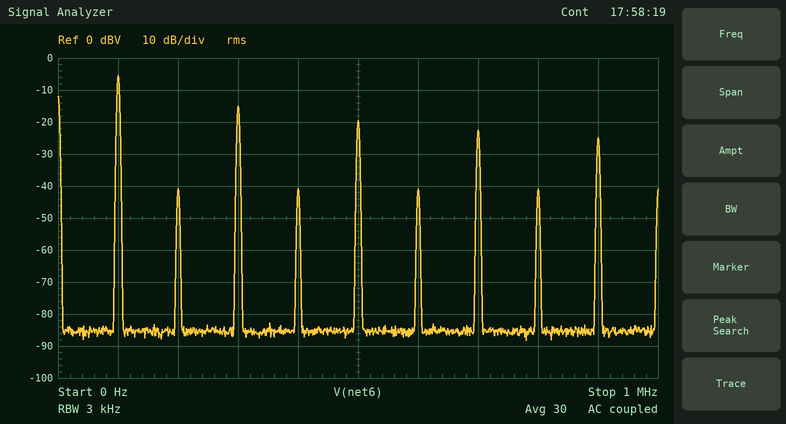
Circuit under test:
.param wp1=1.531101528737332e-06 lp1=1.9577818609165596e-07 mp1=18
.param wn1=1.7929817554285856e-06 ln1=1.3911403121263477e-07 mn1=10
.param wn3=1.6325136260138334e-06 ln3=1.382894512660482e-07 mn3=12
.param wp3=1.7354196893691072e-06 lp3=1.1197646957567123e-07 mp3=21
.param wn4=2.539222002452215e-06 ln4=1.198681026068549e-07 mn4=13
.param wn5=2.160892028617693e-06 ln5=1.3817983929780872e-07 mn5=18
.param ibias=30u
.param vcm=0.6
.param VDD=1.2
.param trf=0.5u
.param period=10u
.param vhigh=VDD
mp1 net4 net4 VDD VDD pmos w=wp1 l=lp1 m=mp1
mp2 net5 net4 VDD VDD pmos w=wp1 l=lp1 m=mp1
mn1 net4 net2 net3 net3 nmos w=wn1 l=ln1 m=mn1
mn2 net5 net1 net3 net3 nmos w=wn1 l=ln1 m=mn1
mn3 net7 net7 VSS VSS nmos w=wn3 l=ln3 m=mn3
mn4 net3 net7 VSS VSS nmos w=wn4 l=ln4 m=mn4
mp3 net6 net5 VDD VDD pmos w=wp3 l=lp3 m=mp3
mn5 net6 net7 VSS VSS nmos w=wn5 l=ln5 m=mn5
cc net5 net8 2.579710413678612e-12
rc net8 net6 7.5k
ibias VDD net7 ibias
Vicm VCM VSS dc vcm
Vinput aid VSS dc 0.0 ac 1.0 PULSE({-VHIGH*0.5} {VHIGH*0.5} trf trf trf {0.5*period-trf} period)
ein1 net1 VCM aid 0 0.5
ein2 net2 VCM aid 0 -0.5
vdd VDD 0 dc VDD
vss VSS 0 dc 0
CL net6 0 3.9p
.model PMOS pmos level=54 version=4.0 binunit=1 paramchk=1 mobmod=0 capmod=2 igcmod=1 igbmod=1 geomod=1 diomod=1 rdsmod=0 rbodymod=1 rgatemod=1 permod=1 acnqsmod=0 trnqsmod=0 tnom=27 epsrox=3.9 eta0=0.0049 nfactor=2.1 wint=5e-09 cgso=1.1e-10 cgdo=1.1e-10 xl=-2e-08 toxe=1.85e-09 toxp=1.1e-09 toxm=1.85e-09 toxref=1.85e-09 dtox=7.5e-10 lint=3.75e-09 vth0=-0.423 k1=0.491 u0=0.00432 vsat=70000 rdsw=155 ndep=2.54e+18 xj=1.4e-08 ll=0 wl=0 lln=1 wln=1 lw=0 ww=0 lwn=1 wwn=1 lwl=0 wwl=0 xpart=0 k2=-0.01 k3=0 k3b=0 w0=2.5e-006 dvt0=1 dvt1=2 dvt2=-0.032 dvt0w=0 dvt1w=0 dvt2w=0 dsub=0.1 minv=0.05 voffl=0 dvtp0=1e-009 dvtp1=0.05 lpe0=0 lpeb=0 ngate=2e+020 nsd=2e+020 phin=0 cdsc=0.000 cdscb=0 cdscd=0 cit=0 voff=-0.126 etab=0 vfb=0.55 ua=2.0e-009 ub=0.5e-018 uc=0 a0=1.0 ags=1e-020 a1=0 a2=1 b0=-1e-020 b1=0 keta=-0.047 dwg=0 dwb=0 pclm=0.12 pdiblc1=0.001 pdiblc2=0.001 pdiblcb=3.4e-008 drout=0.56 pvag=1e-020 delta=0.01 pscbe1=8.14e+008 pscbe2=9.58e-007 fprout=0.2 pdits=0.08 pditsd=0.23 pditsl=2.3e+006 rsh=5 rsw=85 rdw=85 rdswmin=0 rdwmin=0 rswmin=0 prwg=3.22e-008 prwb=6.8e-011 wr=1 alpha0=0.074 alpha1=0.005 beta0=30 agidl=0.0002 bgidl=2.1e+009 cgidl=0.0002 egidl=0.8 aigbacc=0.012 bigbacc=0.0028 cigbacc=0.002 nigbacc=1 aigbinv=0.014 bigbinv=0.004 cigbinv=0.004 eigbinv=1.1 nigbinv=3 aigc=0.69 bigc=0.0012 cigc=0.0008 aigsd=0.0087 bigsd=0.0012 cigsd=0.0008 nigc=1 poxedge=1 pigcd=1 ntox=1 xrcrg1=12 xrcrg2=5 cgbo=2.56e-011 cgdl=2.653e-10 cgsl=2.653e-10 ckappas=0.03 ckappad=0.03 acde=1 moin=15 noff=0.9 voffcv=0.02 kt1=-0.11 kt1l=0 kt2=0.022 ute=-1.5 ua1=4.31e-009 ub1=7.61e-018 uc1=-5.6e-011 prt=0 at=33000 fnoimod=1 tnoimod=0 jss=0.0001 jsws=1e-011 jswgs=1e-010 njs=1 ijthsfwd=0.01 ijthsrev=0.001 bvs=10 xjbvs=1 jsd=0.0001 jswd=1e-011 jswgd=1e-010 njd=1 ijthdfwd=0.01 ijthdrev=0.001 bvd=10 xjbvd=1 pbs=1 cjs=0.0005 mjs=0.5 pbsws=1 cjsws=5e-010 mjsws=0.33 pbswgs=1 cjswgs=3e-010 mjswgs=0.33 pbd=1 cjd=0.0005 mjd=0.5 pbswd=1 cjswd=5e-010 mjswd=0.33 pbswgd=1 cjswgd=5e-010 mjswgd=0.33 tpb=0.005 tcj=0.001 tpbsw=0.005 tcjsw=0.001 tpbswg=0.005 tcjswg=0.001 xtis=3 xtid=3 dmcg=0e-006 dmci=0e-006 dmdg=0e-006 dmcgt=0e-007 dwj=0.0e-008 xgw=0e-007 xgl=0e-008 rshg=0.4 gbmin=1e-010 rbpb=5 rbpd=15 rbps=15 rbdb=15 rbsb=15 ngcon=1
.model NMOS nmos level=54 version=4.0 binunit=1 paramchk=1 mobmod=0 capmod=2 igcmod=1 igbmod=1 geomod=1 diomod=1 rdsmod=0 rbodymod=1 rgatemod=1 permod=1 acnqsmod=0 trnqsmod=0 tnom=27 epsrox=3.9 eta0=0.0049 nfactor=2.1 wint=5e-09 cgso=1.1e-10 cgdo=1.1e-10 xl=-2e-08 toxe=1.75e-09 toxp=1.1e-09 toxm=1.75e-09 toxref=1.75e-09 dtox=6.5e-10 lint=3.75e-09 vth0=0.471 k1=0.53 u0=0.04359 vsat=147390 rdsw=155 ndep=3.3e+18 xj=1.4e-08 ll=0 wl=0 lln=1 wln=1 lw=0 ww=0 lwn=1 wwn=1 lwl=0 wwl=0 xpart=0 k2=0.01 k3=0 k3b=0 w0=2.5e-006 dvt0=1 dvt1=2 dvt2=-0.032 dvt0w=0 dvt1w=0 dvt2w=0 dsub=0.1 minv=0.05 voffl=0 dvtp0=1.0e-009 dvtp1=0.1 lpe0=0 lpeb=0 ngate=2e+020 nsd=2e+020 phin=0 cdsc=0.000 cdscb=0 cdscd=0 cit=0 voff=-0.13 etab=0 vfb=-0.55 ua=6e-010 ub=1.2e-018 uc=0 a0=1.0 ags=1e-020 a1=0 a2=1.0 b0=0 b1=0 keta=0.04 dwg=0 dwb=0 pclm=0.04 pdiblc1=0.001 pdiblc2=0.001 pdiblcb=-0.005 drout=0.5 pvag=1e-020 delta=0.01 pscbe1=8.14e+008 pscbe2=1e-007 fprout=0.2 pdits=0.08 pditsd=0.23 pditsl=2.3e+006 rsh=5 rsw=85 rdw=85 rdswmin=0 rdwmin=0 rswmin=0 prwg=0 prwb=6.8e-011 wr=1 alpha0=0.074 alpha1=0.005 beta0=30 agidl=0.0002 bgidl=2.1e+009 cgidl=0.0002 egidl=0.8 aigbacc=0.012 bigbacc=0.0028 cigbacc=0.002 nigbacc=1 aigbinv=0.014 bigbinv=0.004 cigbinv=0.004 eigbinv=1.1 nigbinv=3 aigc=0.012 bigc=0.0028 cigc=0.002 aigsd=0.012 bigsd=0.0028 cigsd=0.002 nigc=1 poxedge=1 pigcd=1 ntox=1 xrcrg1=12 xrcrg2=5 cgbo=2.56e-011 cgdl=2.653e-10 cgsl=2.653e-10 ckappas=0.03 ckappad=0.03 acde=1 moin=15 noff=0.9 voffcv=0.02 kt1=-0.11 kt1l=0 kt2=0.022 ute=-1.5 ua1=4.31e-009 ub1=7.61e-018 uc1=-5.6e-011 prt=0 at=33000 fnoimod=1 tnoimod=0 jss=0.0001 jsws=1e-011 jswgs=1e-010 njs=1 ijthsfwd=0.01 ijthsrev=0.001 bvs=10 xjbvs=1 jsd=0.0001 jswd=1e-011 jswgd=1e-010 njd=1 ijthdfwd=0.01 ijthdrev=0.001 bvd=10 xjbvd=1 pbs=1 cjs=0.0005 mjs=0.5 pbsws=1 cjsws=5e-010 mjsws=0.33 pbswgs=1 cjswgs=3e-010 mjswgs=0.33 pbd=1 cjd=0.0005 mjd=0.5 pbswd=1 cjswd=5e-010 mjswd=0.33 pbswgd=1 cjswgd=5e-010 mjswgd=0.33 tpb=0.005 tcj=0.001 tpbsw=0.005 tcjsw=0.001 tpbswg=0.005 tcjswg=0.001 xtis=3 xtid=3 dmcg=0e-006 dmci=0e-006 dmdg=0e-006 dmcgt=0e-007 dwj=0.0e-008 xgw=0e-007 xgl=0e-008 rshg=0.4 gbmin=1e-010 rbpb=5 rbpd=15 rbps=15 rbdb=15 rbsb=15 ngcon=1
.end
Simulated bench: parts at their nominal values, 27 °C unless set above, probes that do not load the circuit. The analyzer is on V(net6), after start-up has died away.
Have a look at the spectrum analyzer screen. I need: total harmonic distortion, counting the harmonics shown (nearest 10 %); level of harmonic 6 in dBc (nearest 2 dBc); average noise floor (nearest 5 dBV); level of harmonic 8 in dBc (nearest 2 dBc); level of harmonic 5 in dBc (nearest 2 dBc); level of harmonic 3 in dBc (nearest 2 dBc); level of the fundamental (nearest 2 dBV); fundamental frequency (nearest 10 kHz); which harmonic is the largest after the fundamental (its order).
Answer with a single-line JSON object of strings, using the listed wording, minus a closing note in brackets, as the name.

{"total harmonic distortion, counting the harmonics shown": "40 %", "level of harmonic 6 in dBc": "-36 dBc", "average noise floor": "-85 dBV", "level of harmonic 8 in dBc": "-36 dBc", "level of harmonic 5 in dBc": "-14 dBc", "level of harmonic 3 in dBc": "-10 dBc", "level of the fundamental": "-6 dBV", "fundamental frequency": "100 kHz", "which harmonic is the largest after the fundamental": "3"}
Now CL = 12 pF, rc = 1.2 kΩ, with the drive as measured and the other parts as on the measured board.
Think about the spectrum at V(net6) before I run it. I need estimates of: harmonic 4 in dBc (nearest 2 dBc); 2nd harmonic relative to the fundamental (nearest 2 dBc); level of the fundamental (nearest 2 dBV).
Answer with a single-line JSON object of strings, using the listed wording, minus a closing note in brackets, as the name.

{"harmonic 4 in dBc": "-28 dBc", "2nd harmonic relative to the fundamental": "-28 dBc", "level of the fundamental": "-6 dBV"}
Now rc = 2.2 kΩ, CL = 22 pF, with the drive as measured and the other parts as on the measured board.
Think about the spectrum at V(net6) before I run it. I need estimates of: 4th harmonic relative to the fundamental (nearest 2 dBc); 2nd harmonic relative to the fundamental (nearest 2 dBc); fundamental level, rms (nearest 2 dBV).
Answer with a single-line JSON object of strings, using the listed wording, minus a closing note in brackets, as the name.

{"4th harmonic relative to the fundamental": "-24 dBc", "2nd harmonic relative to the fundamental": "-24 dBc", "fundamental level, rms": "-6 dBV"}
